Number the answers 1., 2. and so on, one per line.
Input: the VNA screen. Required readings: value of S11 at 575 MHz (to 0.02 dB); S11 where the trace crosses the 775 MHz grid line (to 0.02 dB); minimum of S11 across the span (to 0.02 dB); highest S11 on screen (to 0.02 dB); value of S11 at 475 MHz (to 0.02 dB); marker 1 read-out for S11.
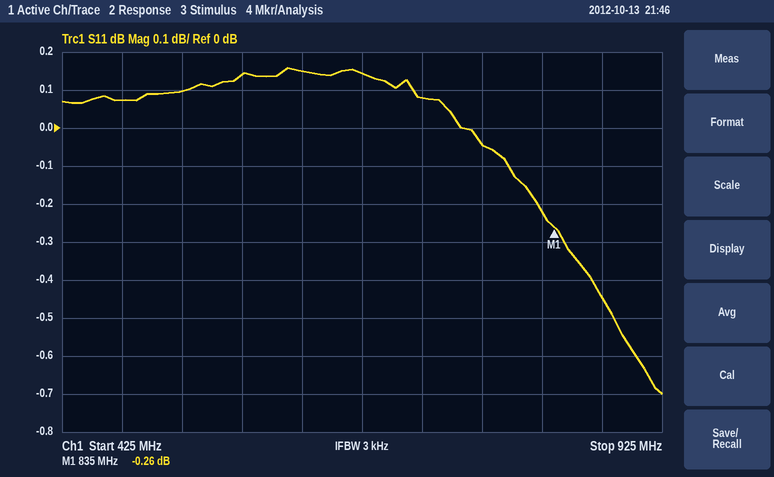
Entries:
1. 0.14 dB
2. -0.04 dB
3. -0.70 dB
4. 0.16 dB
5. 0.08 dB
6. -0.26 dB
